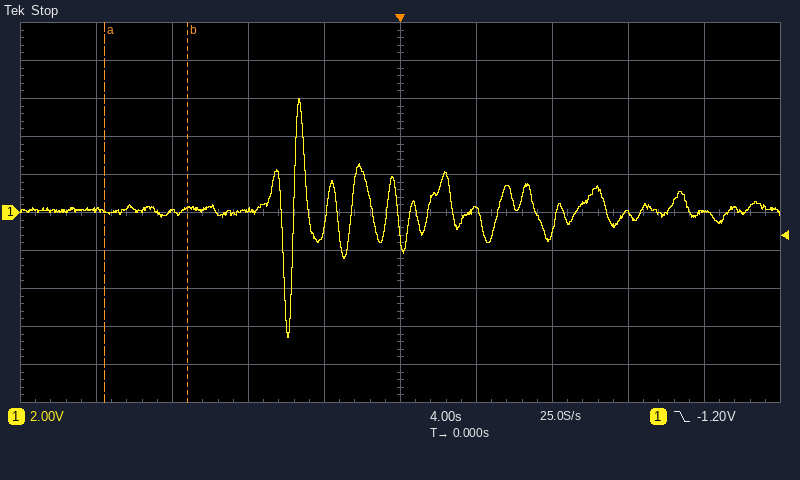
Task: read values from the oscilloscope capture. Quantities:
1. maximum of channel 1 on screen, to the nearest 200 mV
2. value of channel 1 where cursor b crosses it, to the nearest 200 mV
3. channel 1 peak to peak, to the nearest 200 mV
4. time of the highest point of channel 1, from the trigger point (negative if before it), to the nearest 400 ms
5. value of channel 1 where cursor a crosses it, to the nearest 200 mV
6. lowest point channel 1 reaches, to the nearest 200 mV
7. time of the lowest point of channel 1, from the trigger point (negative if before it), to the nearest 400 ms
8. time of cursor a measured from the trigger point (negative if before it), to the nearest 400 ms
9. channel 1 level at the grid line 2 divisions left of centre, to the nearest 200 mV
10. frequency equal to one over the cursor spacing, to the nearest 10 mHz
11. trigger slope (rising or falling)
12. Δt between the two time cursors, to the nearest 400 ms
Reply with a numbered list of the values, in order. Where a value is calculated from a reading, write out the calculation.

1. 6.0 V
2. 200 mV
3. 6.0 V − (-6.6 V) = 12.6 V
4. -5.2 s
5. 0.0 V
6. -6.6 V
7. -6.0 s
8. -15.6 s
9. 200 mV
10. 1 / 4.4 s ≈ 230 mHz
11. falling
12. 4.4 s
